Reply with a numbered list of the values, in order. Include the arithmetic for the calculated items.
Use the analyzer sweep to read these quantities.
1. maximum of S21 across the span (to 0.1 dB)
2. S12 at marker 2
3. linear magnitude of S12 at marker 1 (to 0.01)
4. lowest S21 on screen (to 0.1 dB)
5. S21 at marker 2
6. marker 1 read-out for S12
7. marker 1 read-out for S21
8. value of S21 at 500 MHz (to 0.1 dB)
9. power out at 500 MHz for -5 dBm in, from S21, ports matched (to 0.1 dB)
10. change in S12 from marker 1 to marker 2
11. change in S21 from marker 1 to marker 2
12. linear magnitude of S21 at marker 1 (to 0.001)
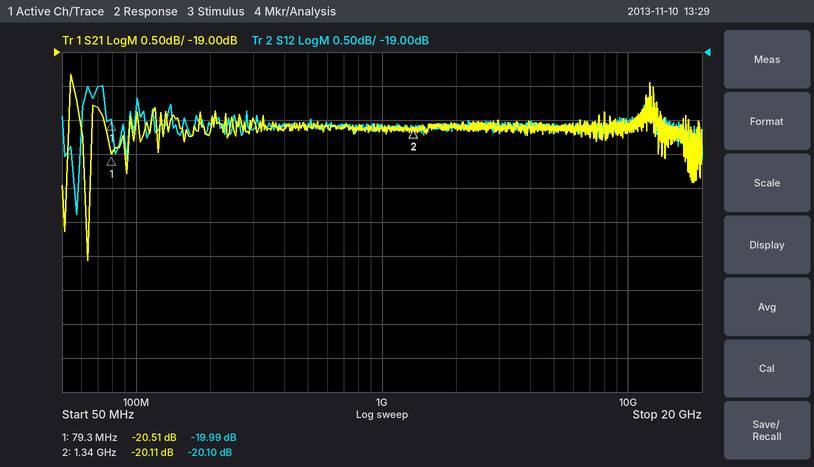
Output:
1. -19.3 dB
2. -20.10 dB
3. 10^(-19.99/20) ≈ 0.10
4. -22.1 dB
5. -20.11 dB
6. -19.99 dB
7. -20.51 dB
8. -20.1 dB
9. -5 dBm + (-20.1 dB) = -25.1 dBm
10. -20.1 − (-19.99) = -0.11 dB
11. -20.11 − (-20.51) = 0.40 dB
12. 10^(-20.51/20) ≈ 0.094
